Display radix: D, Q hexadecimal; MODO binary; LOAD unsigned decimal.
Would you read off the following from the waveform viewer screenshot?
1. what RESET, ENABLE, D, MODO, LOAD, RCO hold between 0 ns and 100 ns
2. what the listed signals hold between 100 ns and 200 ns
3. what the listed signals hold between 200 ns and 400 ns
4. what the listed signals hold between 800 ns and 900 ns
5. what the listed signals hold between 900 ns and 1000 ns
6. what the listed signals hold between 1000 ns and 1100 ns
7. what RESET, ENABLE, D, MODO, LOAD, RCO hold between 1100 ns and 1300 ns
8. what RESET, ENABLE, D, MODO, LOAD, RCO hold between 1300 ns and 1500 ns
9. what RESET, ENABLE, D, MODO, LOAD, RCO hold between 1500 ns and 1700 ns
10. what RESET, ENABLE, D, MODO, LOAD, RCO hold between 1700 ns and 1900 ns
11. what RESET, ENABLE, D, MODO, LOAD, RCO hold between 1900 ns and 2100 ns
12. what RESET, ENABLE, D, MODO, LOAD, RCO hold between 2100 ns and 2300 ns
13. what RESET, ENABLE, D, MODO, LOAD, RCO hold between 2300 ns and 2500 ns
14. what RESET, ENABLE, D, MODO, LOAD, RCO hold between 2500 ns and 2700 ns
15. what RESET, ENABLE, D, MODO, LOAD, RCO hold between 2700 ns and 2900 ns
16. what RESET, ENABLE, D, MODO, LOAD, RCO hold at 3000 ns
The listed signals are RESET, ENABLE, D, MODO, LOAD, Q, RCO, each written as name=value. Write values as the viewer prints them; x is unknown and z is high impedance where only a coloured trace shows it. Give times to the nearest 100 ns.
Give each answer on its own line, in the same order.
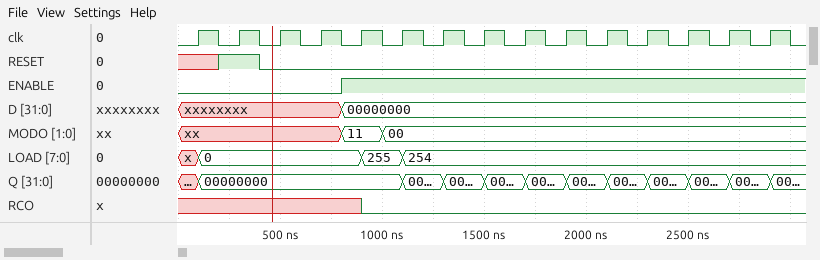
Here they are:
RESET=x, ENABLE=0, D=xxxxxxxx, MODO=xx, LOAD=x, RCO=x
RESET=x, ENABLE=0, D=xxxxxxxx, MODO=xx, LOAD=0, Q=00000000, RCO=x
RESET=1, ENABLE=0, D=xxxxxxxx, MODO=xx, LOAD=0, Q=00000000, RCO=x
RESET=0, ENABLE=1, D=00000000, MODO=11, LOAD=0, Q=00000000, RCO=x
RESET=0, ENABLE=1, D=00000000, MODO=11, LOAD=255, Q=00000000, RCO=0
RESET=0, ENABLE=1, D=00000000, MODO=00, LOAD=255, Q=00000000, RCO=0
RESET=0, ENABLE=1, D=00000000, MODO=00, LOAD=254, RCO=0
RESET=0, ENABLE=1, D=00000000, MODO=00, LOAD=254, RCO=0
RESET=0, ENABLE=1, D=00000000, MODO=00, LOAD=254, RCO=0
RESET=0, ENABLE=1, D=00000000, MODO=00, LOAD=254, RCO=0
RESET=0, ENABLE=1, D=00000000, MODO=00, LOAD=254, RCO=0
RESET=0, ENABLE=1, D=00000000, MODO=00, LOAD=254, RCO=0
RESET=0, ENABLE=1, D=00000000, MODO=00, LOAD=254, RCO=0
RESET=0, ENABLE=1, D=00000000, MODO=00, LOAD=254, RCO=0
RESET=0, ENABLE=1, D=00000000, MODO=00, LOAD=254, RCO=0
RESET=0, ENABLE=1, D=00000000, MODO=00, LOAD=254, RCO=0
